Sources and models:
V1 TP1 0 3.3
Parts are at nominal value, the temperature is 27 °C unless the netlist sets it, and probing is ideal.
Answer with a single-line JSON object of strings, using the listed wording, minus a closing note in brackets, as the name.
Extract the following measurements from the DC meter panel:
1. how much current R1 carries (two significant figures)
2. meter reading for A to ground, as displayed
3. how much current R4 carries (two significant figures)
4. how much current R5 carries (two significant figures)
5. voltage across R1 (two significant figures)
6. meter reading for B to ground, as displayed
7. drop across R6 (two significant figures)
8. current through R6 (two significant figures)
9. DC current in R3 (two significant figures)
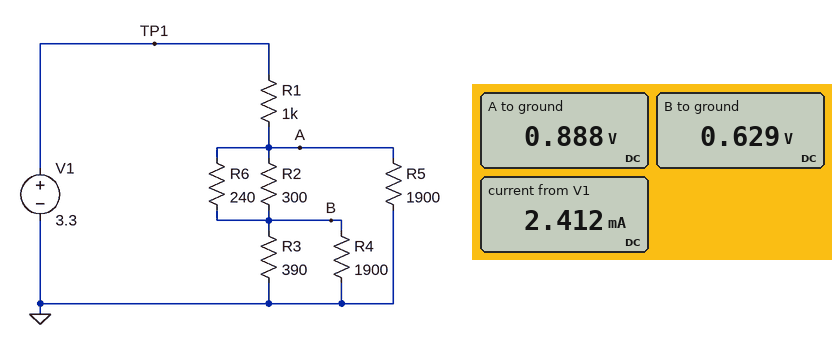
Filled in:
{"how much current R1 carries": "2.4 mA", "meter reading for A to ground, as displayed": "0.888 V", "how much current R4 carries": "330 µA", "how much current R5 carries": "470 µA", "voltage across R1": "2.4 V", "meter reading for B to ground, as displayed": "0.629 V", "drop across R6": "260 mV", "current through R6": "1.1 mA", "DC current in R3": "1.6 mA"}
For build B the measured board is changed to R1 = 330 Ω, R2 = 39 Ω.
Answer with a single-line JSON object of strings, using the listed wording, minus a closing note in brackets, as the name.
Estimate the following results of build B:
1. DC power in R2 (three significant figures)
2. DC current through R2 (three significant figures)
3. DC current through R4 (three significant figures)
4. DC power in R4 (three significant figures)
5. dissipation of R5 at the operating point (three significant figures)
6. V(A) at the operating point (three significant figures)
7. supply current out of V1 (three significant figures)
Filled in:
{"DC power in R2": "560 µW", "DC current through R2": "3.79 mA", "DC current through R4": "750 µA", "DC power in R4": "1.07 mW", "dissipation of R5 at the operating point": "1.30 mW", "V(A) at the operating point": "1.57 V", "supply current out of V1": "5.23 mA"}
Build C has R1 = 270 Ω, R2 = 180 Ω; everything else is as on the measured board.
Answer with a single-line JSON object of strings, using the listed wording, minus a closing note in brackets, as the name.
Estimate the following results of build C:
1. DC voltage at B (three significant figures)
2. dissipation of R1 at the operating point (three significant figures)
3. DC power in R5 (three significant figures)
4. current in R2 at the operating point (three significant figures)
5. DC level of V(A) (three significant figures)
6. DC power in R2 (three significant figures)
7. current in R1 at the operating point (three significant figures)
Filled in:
{"DC voltage at B": "1.41 V", "dissipation of R1 at the operating point": "7.69 mW", "DC power in R5": "1.82 mW", "current in R2 at the operating point": "2.49 mA", "DC level of V(A)": "1.86 V", "DC power in R2": "1.12 mW", "current in R1 at the operating point": "5.34 mA"}
